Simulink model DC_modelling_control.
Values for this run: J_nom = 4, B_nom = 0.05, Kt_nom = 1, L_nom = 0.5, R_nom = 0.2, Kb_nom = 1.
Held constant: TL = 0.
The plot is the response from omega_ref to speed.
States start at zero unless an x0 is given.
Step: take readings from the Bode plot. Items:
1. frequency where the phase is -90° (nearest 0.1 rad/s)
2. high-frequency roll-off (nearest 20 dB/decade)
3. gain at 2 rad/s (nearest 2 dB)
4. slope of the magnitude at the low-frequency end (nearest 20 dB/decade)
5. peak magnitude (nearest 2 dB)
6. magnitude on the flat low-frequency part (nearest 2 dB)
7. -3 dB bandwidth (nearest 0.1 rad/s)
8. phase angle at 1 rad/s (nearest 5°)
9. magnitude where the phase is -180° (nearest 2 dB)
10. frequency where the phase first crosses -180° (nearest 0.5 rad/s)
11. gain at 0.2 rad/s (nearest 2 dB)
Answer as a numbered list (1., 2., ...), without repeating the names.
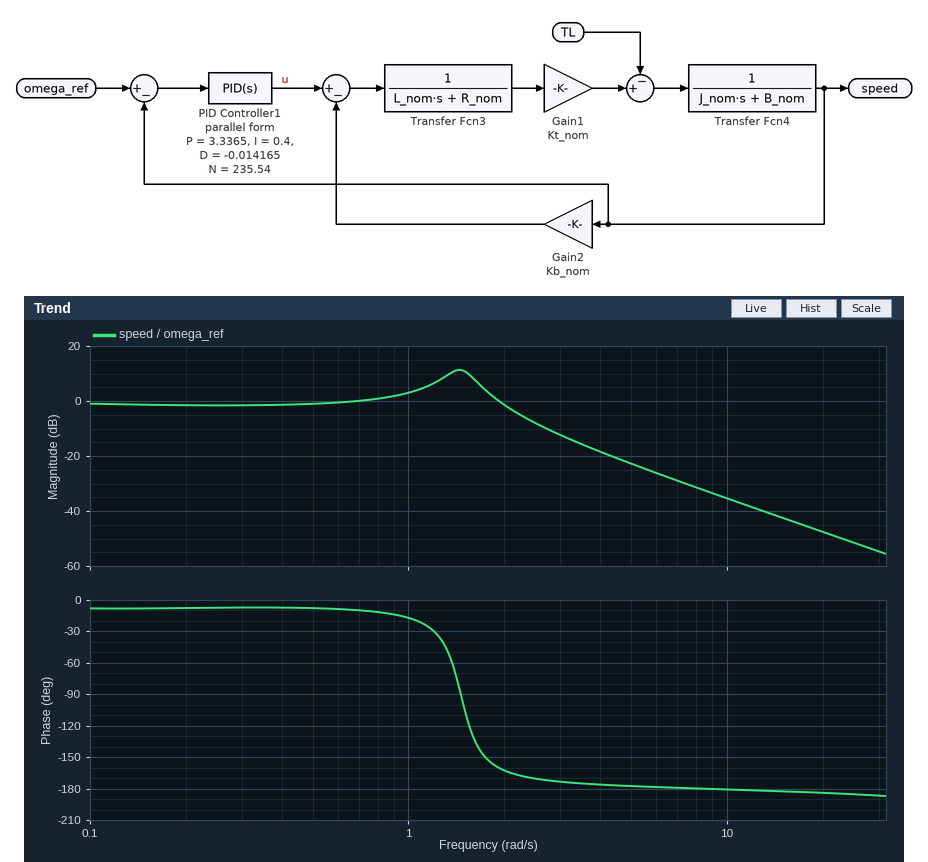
1. 1.5 rad/s
2. -40 dB/decade
3. -2 dB
4. 0 dB/decade
5. 12 dB
6. -2 dB
7. 2.2 rad/s
8. -15°
9. -32 dB
10. 8.5 rad/s
11. -2 dB
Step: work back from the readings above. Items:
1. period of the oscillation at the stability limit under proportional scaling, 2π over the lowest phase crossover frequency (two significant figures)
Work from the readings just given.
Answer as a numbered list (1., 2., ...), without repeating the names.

1. 0.74 s
